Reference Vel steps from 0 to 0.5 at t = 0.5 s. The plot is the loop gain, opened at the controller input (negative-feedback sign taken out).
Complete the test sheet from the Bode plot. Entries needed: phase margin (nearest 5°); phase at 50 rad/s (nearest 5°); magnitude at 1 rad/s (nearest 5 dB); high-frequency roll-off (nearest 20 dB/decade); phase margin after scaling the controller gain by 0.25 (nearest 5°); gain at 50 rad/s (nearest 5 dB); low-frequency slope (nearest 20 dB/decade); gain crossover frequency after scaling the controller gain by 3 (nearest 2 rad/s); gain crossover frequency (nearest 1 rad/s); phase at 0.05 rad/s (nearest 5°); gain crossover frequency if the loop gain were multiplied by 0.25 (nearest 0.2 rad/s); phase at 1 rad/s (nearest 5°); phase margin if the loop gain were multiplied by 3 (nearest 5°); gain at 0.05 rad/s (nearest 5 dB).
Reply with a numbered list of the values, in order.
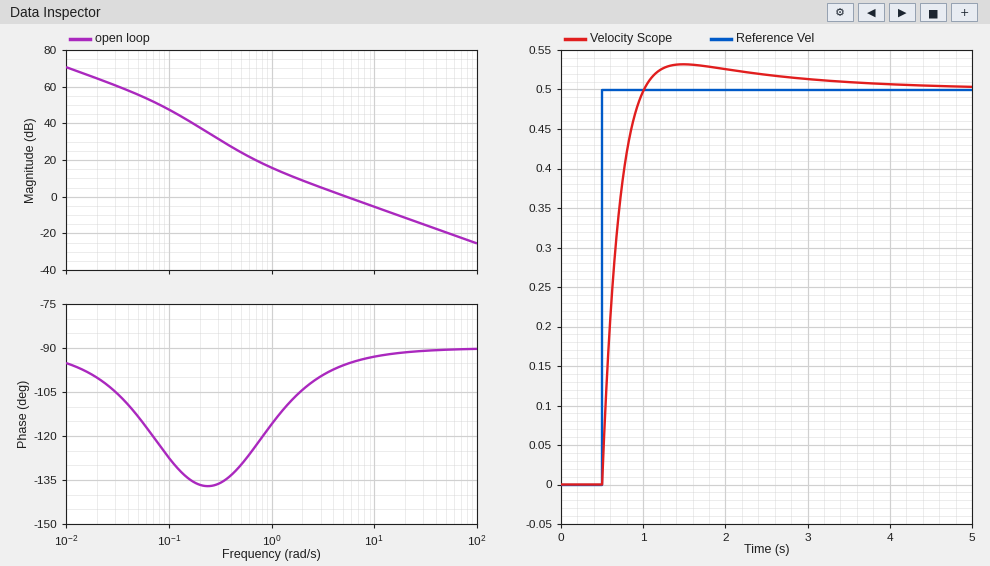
1. 85°
2. -90°
3. 15 dB
4. -20 dB/decade
5. 70°
6. -20 dB
7. -20 dB/decade
8. 16 rad/s
9. 5 rad/s
10. -115°
11. 1.4 rad/s
12. -115°
13. 90°
14. 55 dB
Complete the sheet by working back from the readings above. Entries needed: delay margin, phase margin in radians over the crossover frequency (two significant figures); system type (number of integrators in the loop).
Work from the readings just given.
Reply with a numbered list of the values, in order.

1. 0.30 s
2. 1
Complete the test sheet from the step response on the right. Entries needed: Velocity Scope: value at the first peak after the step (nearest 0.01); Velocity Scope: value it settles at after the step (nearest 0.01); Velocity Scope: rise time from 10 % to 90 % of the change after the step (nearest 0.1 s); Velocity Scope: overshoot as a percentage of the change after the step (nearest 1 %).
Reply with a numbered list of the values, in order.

1. 0.53
2. 0.50
3. 0.3 s
4. 6 %
